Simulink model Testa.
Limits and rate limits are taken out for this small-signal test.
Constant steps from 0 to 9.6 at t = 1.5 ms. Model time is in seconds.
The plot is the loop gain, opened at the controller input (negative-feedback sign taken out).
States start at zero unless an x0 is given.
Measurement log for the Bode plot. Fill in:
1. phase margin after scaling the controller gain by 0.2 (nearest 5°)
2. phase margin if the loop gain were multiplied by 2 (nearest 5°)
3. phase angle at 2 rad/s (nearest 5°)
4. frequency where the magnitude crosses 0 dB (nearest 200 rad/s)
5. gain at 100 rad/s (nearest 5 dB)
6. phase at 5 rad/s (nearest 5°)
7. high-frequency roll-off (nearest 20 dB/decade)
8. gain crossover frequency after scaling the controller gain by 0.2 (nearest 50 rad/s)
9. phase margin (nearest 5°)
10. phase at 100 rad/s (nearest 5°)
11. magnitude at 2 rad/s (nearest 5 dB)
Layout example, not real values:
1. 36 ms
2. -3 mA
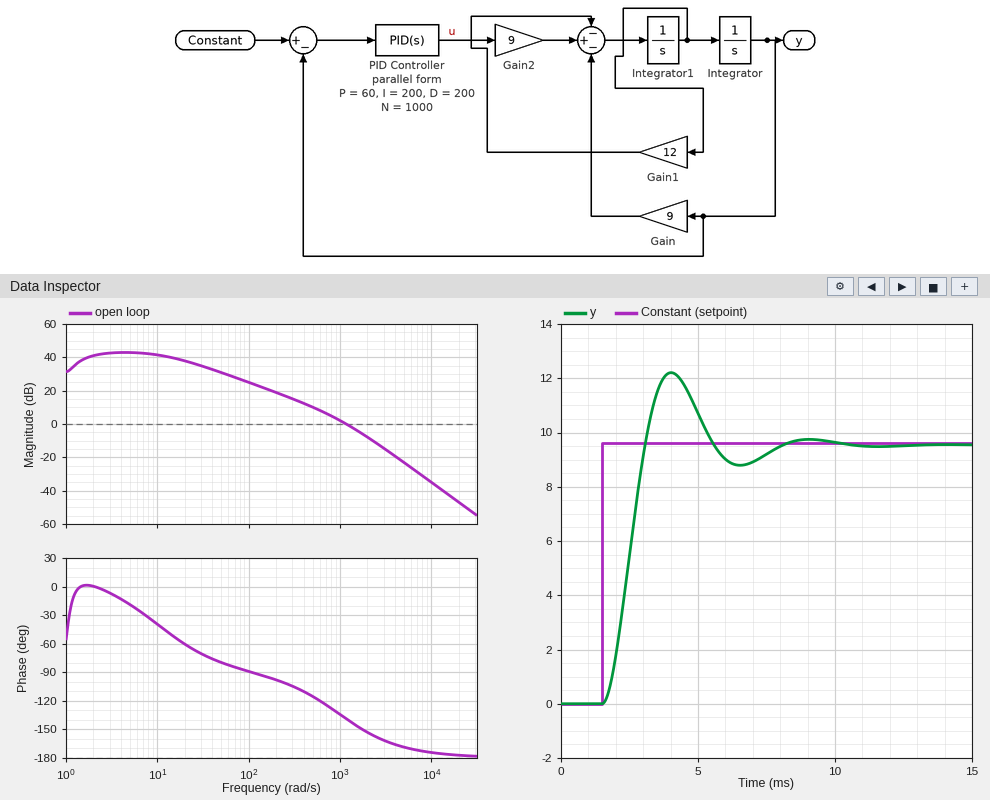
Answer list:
1. 75°
2. 30°
3. 0°
4. 1200 rad/s
5. 25 dB
6. -20°
7. -40 dB/decade
8. 350 rad/s
9. 40°
10. -90°
11. 40 dB
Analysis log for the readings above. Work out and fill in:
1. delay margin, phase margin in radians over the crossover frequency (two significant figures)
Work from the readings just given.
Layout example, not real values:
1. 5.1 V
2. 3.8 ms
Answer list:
1. 0.00058 s
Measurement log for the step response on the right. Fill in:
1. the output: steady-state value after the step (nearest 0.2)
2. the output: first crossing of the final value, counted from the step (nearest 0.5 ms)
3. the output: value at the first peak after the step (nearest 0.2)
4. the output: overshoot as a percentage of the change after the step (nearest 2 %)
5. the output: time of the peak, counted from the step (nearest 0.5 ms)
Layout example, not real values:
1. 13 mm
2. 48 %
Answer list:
1. 9.6
2. 1.5 ms
3. 12.2
4. 28 %
5. 2.5 ms
